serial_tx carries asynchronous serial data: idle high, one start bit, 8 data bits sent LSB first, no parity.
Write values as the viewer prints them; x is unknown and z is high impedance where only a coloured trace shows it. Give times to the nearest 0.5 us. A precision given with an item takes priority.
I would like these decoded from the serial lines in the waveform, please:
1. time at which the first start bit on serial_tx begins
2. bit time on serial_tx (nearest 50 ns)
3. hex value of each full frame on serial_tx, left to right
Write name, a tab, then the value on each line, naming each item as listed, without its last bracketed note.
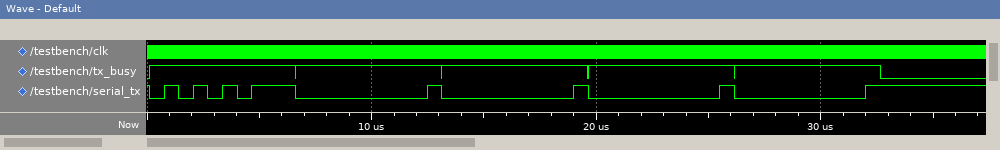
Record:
time at which the first start bit on serial_tx begins	0 us
bit time on serial_tx	650 ns
hex value of each full frame on serial_tx, left to right	D5, 00, 00, 00, 00
